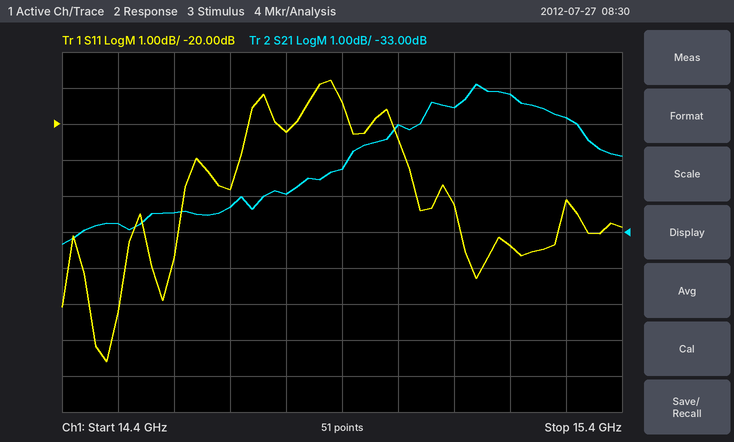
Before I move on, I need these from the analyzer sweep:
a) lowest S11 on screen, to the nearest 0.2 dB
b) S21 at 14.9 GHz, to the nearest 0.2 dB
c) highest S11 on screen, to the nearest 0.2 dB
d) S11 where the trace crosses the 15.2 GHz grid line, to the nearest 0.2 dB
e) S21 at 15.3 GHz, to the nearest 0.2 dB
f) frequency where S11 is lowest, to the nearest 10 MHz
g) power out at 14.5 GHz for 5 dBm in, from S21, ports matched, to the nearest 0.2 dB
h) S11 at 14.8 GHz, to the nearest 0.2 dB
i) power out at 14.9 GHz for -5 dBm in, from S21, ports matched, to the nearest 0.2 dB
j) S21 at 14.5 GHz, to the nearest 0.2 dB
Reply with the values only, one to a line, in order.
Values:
-26.6 dB
-31.2 dB
-18.8 dB
-23.4 dB
-29.8 dB
14.48 GHz
-27.8 dBm
-20.2 dB
-36.2 dBm
-32.8 dB
